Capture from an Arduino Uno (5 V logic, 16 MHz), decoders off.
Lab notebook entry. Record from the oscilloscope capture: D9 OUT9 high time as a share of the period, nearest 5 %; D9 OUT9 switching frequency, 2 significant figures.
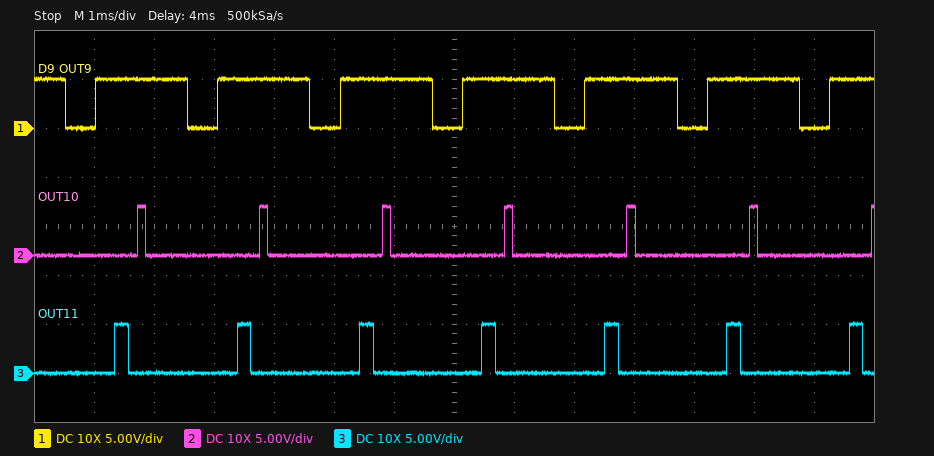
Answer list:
75 %
490 Hz
